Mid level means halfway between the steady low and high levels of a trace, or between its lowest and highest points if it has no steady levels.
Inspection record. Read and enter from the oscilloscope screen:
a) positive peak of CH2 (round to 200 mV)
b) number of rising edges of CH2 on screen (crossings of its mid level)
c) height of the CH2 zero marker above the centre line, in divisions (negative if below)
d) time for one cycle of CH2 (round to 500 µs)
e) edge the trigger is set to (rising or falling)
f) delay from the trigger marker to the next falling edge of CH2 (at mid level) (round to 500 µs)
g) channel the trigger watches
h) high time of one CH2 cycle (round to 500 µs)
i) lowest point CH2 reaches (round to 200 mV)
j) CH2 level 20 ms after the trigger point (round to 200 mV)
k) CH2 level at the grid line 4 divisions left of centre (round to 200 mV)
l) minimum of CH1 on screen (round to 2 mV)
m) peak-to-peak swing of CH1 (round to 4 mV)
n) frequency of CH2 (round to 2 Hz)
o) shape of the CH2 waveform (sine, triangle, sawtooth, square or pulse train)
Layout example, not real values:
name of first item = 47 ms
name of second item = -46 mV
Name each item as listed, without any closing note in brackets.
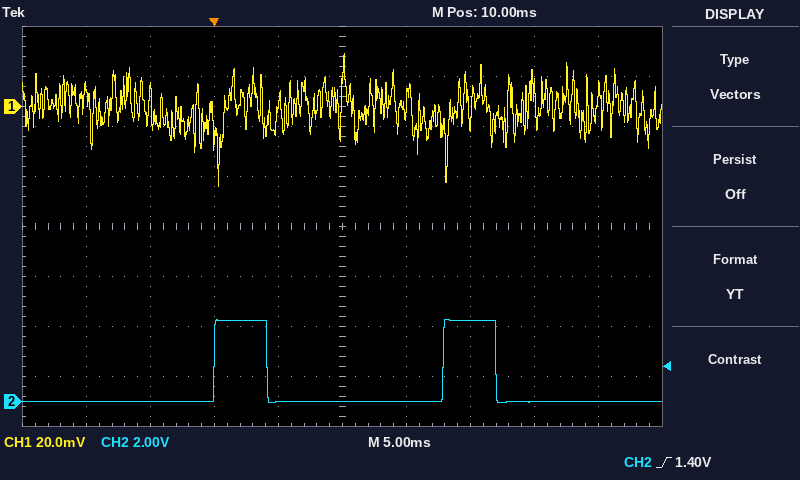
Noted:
positive peak of CH2 = 3.2 V
number of rising edges of CH2 on screen = 2
height of the CH2 zero marker above the centre line, in divisions = -3.5 div
time for one cycle of CH2 = 18.0 ms
edge the trigger is set to = rising
delay from the trigger marker to the next falling edge of CH2 (at mid level) = 4.0 ms
channel the trigger watches = CH2
high time of one CH2 cycle = 4.0 ms
lowest point CH2 reaches = 0.0 V
CH2 level 20 ms after the trigger point = 3.2 V
CH2 level at the grid line 4 divisions left of centre = 0.0 V
minimum of CH1 on screen = -32 mV
peak-to-peak swing of CH1 = 52 mV
frequency of CH2 = 56 Hz
shape of the CH2 waveform = pulse train
